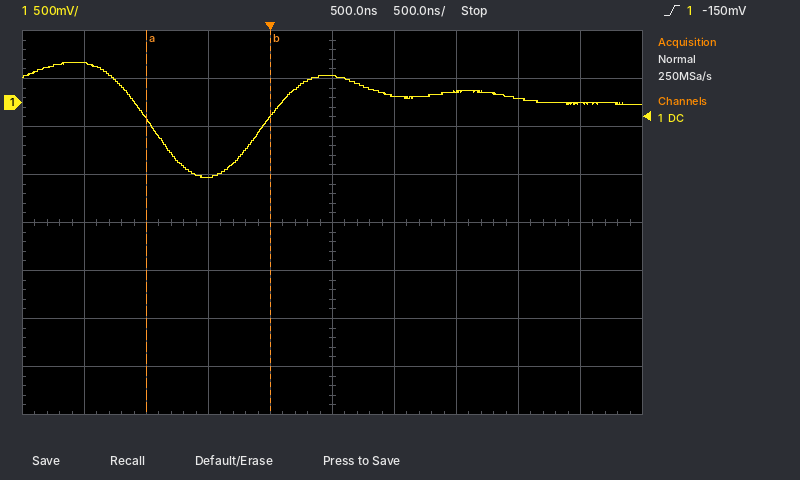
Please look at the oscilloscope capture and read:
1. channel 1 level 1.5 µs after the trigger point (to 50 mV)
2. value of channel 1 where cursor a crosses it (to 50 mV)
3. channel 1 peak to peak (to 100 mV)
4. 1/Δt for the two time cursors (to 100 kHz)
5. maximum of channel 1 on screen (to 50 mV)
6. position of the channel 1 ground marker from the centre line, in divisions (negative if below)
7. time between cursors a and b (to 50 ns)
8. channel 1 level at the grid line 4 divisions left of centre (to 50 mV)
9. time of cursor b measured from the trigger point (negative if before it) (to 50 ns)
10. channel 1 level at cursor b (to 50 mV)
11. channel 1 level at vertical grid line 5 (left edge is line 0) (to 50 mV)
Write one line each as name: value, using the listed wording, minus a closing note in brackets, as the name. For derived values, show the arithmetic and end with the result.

channel 1 level 1.5 µs after the trigger point: 100 mV
value of channel 1 where cursor a crosses it: -150 mV
channel 1 peak to peak: 1.20 V
1/Δt for the two time cursors: 1 / 1.00 µs ≈ 1.0 MHz
maximum of channel 1 on screen: 400 mV
position of the channel 1 ground marker from the centre line, in divisions: +2.5 div
time between cursors a and b: 1.00 µs
channel 1 level at the grid line 4 divisions left of centre: 400 mV
time of cursor b measured from the trigger point (negative if before it): 0 ns
channel 1 level at cursor b: -150 mV
channel 1 level at vertical grid line 5 (left edge is line 0): 300 mV
